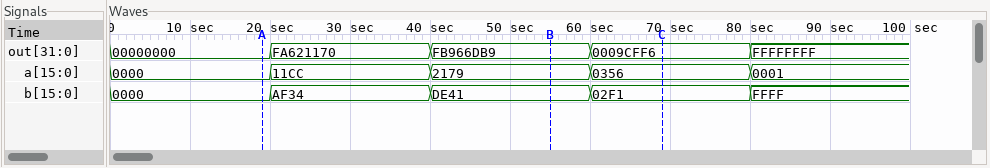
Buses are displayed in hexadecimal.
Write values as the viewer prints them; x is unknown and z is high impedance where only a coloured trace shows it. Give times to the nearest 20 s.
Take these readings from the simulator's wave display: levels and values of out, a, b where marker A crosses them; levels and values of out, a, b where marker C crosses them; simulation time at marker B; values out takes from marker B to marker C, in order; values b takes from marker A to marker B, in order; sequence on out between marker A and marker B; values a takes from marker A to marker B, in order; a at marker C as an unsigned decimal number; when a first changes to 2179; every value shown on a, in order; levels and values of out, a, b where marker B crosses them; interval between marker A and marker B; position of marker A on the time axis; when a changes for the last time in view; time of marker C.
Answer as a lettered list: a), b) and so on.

a) out=00000000, a=0000, b=0000
b) out=0009CFF6, a=0356, b=02F1
c) 60 s
d) FB966DB9, 0009CFF6
e) 0000, AF34, DE41
f) 00000000, FA621170, FB966DB9
g) 0000, 11CC, 2179
h) 854
i) 40 s
j) 0000, 11CC, 2179, 0356, 0001
k) out=FB966DB9, a=2179, b=DE41
l) 40 s
m) 20 s
n) 80 s
o) 60 s
